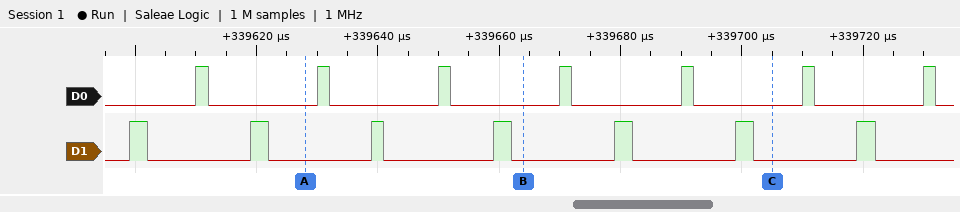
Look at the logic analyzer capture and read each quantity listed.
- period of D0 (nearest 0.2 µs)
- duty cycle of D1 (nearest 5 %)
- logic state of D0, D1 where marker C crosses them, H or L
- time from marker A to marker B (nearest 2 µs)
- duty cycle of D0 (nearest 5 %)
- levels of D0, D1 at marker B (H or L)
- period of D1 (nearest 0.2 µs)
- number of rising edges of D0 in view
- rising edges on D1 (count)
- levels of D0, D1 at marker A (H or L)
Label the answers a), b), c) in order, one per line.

a) 20 µs
b) 15 %
c) D0=L, D1=L
d) 36 µs
e) 10 %
f) D0=L, D1=L
g) 20 µs
h) 7
i) 7
j) D0=L, D1=L
